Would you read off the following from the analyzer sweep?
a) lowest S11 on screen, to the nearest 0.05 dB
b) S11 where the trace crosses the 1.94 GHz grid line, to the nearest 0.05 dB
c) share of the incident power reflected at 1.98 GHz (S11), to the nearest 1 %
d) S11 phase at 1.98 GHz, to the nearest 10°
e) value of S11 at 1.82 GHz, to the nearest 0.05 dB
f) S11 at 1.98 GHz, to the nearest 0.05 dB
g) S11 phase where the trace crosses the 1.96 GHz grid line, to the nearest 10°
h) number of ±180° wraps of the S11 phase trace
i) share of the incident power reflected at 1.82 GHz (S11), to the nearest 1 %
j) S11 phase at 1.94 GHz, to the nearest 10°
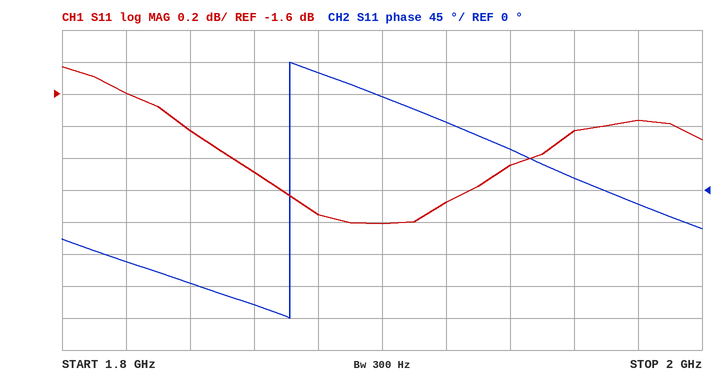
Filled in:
-2.40 dB
-2.05 dB
67 %
-20°
-1.60 dB
-1.75 dB
20°
1
69 %
60°
